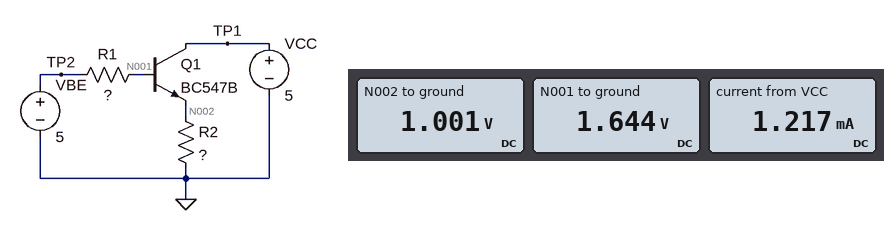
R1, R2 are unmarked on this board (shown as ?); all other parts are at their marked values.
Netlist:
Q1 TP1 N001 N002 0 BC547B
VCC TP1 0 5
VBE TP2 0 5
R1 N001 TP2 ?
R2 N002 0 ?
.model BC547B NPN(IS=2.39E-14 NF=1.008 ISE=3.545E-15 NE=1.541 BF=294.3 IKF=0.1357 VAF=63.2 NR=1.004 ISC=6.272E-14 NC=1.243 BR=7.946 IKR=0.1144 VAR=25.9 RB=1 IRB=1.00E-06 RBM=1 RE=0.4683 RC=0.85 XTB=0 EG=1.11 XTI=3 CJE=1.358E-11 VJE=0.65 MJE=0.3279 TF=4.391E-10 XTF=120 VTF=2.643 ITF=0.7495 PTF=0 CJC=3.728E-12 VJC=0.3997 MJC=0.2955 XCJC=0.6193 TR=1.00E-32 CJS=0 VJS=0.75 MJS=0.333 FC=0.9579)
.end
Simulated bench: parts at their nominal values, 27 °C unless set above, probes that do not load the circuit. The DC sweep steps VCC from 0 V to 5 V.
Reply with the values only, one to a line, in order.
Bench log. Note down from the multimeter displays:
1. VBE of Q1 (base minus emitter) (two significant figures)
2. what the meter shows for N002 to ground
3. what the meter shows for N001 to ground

640 mV
1.001 V
1.644 V
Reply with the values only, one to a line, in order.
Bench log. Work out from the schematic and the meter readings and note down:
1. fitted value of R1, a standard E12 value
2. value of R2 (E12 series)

820 kΩ
820 Ω
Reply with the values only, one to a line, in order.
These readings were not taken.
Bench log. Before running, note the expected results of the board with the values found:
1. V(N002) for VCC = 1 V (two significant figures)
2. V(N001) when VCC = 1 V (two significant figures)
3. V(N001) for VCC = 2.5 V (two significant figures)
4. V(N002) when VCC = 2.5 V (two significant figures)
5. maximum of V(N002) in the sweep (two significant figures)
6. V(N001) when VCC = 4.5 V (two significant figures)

840 mV
1.5 V
1.6 V
970 mV
1.0 V
1.6 V
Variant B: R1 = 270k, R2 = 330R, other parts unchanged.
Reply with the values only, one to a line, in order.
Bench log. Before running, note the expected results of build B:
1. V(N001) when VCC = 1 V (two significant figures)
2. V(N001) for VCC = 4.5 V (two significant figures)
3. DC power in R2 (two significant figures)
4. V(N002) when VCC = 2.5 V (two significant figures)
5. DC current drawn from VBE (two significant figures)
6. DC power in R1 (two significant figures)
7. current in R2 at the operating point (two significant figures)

1.5 V
1.8 V
4.0 mW
1.1 V
12 µA
38 µW
3.5 mA
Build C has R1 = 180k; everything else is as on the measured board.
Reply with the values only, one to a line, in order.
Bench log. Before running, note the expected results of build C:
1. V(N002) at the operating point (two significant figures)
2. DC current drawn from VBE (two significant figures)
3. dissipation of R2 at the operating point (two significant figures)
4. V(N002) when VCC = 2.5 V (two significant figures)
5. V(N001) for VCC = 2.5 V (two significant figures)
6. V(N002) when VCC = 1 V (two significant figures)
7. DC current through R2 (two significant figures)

2.5 V
10 µA
7.4 mW
2.3 V
3.0 V
930 mV
3.0 mA
